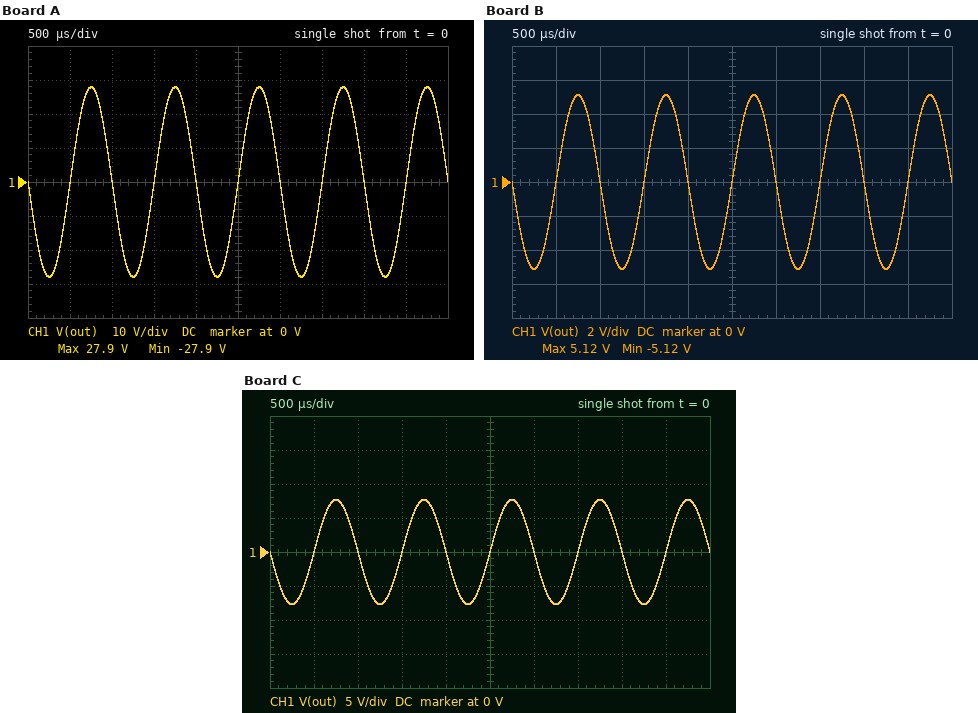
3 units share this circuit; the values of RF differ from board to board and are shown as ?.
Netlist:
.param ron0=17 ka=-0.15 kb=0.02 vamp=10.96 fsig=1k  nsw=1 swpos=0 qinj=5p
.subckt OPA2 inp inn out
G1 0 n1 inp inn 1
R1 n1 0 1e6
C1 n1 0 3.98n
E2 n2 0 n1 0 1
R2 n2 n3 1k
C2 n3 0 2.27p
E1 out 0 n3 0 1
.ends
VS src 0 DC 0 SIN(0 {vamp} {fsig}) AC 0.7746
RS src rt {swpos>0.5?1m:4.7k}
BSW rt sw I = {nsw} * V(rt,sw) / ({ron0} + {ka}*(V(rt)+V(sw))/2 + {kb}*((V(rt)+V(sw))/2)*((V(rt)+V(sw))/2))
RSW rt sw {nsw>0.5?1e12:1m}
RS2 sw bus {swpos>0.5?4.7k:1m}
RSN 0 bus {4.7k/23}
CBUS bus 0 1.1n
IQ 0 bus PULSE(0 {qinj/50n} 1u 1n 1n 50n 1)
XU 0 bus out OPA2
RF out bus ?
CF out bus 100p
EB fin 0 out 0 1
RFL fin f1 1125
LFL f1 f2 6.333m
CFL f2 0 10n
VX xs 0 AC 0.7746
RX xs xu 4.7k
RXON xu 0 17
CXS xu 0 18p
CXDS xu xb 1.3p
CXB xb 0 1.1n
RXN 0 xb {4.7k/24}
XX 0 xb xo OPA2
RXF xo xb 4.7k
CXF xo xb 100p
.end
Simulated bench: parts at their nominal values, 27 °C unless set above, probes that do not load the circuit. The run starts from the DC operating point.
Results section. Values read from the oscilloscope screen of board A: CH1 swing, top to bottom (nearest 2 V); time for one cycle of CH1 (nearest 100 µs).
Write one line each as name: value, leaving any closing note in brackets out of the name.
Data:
CH1 swing, top to bottom: 56 V
time for one cycle of CH1: 1.0 ms
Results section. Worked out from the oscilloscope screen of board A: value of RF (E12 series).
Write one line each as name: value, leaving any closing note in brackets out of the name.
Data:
value of RF: 12 kΩ
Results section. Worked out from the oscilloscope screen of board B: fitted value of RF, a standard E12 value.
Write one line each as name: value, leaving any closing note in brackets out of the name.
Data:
fitted value of RF, a standard E12 value: 2.2 kΩ
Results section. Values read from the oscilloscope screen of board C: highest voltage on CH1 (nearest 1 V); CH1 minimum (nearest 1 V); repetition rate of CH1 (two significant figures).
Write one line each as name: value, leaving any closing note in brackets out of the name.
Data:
highest voltage on CH1: 8 V
CH1 minimum: -8 V
repetition rate of CH1: 1.0 kHz
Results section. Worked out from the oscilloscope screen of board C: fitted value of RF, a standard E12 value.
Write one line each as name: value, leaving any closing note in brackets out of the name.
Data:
fitted value of RF, a standard E12 value: 3.3 kΩ
